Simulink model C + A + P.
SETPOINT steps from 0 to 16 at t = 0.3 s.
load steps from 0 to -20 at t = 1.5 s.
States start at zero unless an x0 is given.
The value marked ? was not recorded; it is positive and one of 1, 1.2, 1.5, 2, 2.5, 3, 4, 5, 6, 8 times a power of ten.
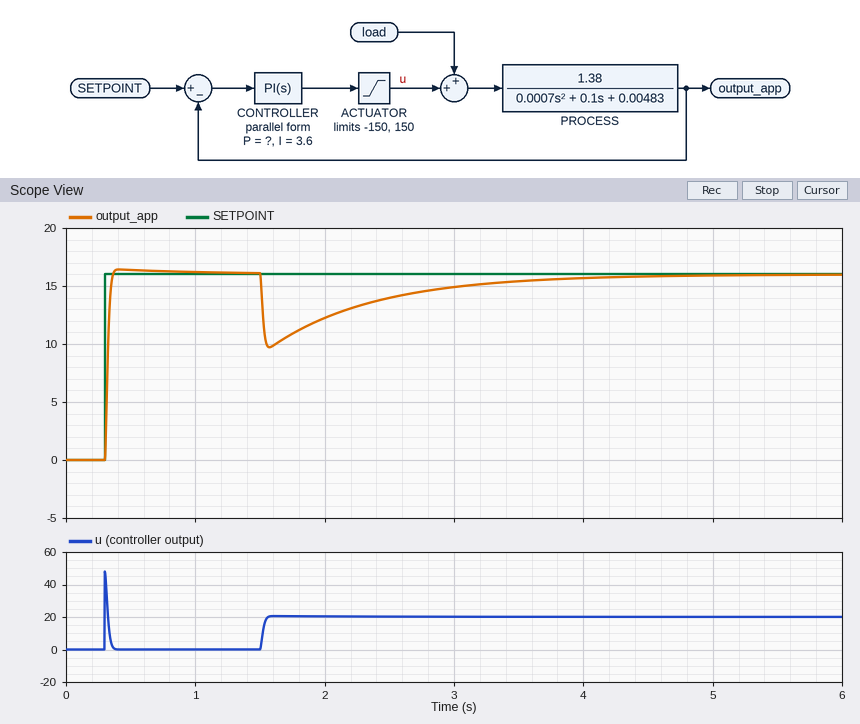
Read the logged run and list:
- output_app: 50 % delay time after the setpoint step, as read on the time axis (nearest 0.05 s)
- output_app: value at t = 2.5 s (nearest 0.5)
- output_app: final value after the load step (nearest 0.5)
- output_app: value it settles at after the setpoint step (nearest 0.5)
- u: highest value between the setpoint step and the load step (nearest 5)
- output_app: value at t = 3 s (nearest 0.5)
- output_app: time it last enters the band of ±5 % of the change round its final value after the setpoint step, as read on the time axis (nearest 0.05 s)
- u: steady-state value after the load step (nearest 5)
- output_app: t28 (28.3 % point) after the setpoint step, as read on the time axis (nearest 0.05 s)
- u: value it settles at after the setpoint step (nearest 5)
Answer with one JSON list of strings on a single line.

["0.30 s", "14.0", "16.0", "16.0", "50", "15.0", "0.35 s", "20", "0.30 s", "0"]
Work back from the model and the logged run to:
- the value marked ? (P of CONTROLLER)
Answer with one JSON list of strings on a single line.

["3"]
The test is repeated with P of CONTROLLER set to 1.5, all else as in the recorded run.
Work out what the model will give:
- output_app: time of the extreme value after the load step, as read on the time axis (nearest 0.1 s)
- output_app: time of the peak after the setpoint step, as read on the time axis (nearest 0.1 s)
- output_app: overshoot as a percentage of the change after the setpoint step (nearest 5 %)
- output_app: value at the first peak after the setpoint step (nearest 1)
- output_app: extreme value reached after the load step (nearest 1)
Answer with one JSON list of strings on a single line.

["1.6 s", "0.5 s", "10 %", "17", "5"]
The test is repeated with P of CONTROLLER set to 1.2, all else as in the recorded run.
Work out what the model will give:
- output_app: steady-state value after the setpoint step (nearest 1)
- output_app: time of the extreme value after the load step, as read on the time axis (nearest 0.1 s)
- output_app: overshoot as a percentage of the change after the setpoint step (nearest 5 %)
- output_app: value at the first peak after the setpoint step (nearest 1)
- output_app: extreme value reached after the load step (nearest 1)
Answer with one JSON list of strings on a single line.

["16", "1.6 s", "10 %", "18", "3"]
